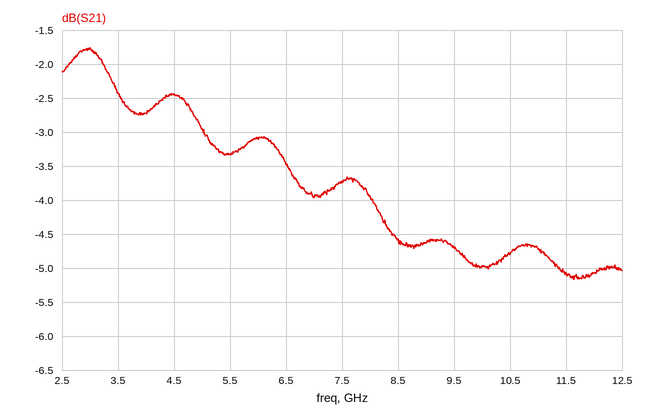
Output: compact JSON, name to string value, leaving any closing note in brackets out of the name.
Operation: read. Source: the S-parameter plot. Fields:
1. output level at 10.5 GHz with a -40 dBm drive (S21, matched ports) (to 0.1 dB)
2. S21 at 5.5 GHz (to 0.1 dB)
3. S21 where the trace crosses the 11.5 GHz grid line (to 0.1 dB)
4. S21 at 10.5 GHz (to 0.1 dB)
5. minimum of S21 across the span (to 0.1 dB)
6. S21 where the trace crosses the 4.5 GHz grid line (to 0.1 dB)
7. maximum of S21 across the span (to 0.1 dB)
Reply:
{"output level at 10.5 GHz with a -40 dBm drive (S21, matched ports)": "-44.8 dBm", "S21 at 5.5 GHz": "-3.3 dB", "S21 where the trace crosses the 11.5 GHz grid line": "-5.1 dB", "S21 at 10.5 GHz": "-4.8 dB", "minimum of S21 across the span": "-5.2 dB", "S21 where the trace crosses the 4.5 GHz grid line": "-2.4 dB", "maximum of S21 across the span": "-1.8 dB"}
